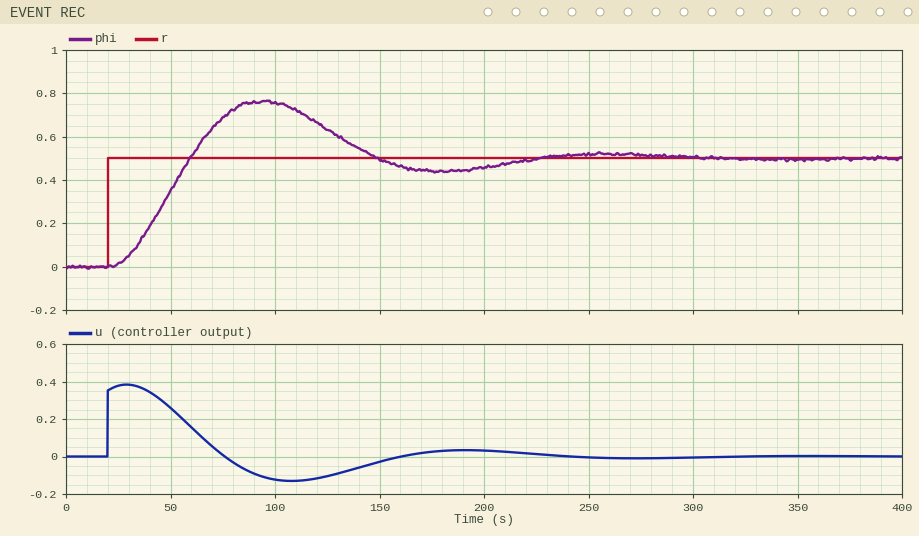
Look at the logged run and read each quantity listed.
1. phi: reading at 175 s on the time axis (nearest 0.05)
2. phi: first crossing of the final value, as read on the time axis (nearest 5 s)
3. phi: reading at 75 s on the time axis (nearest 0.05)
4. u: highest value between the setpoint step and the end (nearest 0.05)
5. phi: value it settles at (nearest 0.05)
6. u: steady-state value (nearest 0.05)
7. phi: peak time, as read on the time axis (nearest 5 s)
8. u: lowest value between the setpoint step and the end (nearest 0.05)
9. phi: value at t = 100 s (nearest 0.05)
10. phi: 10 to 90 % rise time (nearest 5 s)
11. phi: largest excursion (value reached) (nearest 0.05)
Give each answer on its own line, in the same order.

0.45
60 s
0.70
0.40
0.50
0.00
95 s
-0.15
0.75
25 s
0.75
